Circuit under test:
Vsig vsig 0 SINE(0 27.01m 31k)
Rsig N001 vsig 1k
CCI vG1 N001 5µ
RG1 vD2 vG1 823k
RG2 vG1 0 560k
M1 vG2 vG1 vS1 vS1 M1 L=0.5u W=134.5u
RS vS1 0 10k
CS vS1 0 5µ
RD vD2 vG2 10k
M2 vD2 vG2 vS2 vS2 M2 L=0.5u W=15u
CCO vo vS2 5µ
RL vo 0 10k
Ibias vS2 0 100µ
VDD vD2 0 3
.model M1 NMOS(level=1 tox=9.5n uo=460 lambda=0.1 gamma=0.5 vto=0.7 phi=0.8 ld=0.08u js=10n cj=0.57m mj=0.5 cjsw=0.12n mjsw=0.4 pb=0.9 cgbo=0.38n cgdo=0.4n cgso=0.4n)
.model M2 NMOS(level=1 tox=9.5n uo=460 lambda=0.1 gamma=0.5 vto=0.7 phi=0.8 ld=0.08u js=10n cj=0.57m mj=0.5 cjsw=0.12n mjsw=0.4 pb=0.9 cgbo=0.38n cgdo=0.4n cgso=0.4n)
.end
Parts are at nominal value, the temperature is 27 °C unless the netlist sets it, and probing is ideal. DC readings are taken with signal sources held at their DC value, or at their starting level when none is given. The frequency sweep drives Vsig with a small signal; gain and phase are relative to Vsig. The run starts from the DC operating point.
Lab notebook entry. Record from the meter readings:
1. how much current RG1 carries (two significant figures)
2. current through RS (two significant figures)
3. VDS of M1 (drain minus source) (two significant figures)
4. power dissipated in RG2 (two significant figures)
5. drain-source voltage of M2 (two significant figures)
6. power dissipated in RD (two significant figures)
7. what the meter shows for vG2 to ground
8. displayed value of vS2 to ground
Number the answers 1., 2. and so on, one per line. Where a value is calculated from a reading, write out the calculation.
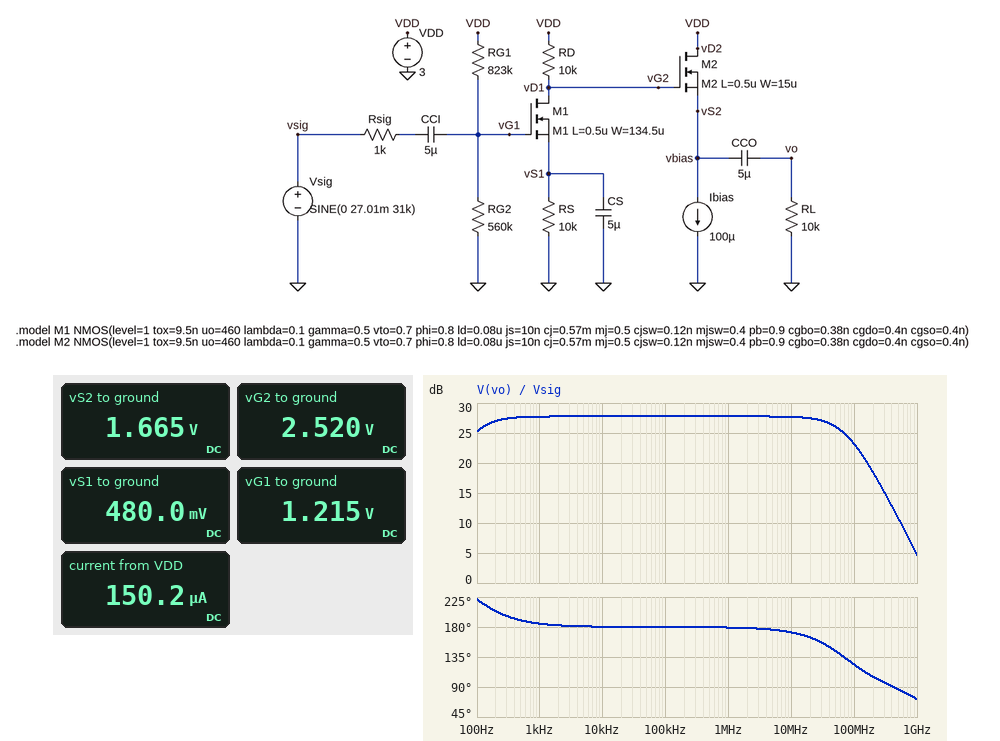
1. (3 V - 1.215 V) / 823 kΩ = 2.2 µA
2. (480 mV) / 10 kΩ = 48 µA
3. 2.52 V - 480 mV = 2.0 V
4. (1.215 V)^2 / 560 kΩ = 2.6 µW
5. 3 V - 1.665 V = 1.3 V
6. (3 V - 2.52 V)^2 / 10 kΩ = 23 µW
7. 2.520 V
8. 1.665 V
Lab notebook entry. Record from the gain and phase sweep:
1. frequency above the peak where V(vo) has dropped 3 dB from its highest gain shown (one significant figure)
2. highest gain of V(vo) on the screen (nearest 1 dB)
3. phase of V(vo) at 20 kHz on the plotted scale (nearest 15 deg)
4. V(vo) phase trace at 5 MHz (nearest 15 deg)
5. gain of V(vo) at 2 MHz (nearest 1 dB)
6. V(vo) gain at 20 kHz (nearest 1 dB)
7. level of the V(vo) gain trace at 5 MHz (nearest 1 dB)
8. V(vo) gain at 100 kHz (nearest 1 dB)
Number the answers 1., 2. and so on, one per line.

1. 70 MHz
2. 28 dB
3. 180 deg
4. 180 deg
5. 28 dB
6. 28 dB
7. 28 dB
8. 28 dB
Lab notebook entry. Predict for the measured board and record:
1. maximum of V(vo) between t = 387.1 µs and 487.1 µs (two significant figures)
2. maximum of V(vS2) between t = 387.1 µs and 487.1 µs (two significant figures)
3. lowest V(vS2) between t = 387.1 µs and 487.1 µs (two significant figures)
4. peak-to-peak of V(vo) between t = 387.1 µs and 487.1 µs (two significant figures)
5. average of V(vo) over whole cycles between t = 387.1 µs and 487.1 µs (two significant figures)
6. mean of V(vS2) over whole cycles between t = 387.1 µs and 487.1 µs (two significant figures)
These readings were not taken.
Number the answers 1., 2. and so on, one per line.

1. 430 mV
2. 2.1 V
3. 870 mV
4. 1.2 V
5. -80 mV
6. 1.6 V
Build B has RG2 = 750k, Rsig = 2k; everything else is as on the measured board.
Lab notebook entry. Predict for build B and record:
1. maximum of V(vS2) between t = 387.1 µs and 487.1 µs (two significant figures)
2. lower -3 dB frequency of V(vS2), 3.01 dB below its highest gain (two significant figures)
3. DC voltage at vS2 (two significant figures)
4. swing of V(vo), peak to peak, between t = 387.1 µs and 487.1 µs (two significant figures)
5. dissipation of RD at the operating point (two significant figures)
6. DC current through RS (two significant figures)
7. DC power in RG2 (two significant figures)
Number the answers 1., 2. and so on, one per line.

1. 2.0 V
2. 100 Hz
3. 1.5 V
4. 1.4 V
5. 47 µW
6. 69 µA
7. 2.7 µW
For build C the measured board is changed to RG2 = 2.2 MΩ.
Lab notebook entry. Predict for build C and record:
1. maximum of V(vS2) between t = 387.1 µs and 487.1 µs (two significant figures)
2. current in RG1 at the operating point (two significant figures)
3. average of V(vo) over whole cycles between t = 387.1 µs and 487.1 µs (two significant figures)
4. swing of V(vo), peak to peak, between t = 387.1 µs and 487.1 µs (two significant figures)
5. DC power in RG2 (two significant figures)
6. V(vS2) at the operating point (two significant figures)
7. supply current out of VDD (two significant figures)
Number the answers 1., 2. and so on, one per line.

1. 1.5 V
2. 990 nA
3. 190 mV
4. 910 mV
5. 2.2 µW
6. 730 mV
7. 240 µA
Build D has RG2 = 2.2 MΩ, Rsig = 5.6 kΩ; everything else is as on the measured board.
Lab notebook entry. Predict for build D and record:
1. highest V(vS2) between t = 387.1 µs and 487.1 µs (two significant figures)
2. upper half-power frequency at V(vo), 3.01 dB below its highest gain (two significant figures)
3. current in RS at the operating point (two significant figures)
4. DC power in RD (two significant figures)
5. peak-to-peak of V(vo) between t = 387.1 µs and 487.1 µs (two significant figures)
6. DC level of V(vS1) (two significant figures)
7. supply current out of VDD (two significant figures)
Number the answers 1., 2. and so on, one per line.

1. 1.5 V
2. 12 MHz
3. 140 µA
4. 200 µW
5. 910 mV
6. 1.4 V
7. 240 µA
